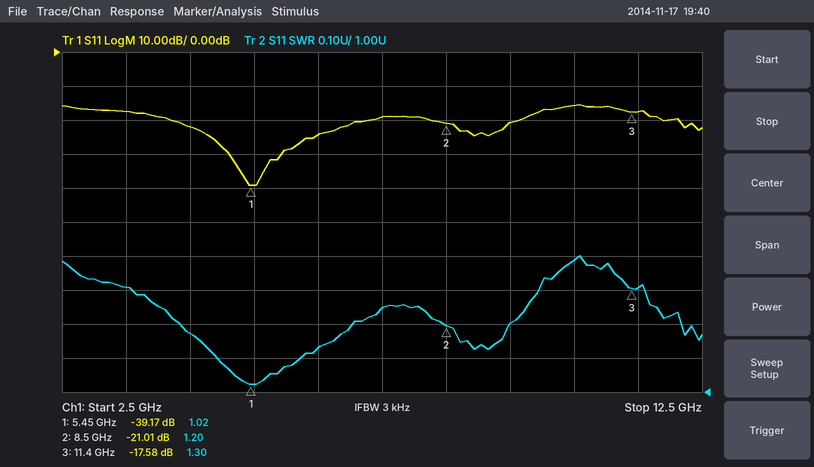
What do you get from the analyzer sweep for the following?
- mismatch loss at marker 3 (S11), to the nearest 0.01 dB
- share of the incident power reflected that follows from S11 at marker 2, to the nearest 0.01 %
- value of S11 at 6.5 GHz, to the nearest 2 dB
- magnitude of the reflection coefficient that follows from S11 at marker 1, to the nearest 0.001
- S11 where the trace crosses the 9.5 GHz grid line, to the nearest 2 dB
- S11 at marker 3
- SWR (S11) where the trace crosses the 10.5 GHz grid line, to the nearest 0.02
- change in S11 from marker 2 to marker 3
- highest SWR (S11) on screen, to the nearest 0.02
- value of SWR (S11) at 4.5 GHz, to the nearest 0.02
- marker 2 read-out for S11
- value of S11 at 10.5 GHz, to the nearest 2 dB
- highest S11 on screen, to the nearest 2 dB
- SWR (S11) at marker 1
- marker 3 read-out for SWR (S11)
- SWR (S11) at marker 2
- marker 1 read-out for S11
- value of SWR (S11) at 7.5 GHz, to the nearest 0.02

0.08 dB
0.79 %
-24 dB
0.011
-20 dB
-17.58 dB
1.38
3.43 dB
1.40
1.18
-21.01 dB
-16 dB
-16 dB
1.02
1.30
1.20
-39.17 dB
1.24
